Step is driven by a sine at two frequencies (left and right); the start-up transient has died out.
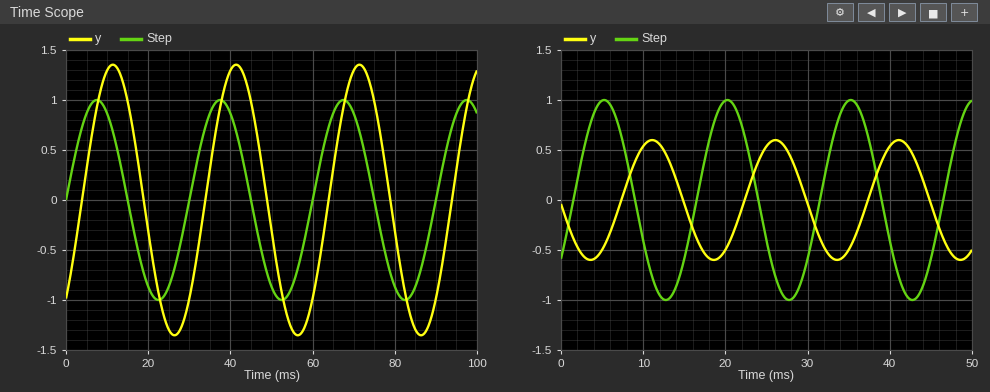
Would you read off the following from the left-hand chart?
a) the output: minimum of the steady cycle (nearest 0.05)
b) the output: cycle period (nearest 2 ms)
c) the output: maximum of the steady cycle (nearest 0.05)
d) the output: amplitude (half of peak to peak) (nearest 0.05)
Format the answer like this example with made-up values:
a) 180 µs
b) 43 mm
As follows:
a) -1.35
b) 30 ms
c) 1.35
d) 1.35
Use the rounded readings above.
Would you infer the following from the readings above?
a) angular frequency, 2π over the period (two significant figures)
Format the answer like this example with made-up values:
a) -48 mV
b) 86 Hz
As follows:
a) 0.21 rad/ms
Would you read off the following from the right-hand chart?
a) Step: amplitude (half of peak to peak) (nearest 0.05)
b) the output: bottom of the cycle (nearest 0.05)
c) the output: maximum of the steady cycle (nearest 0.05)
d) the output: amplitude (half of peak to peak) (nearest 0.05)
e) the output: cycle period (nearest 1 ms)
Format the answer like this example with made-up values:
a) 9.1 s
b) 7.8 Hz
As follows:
a) 1.00
b) -0.60
c) 0.60
d) 0.60
e) 15 ms
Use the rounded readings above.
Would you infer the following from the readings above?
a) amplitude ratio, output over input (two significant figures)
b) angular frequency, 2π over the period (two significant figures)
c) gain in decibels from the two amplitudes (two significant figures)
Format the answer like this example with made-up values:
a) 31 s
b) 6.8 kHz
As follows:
a) 0.60
b) 0.42 rad/ms
c) -4.4 dB
